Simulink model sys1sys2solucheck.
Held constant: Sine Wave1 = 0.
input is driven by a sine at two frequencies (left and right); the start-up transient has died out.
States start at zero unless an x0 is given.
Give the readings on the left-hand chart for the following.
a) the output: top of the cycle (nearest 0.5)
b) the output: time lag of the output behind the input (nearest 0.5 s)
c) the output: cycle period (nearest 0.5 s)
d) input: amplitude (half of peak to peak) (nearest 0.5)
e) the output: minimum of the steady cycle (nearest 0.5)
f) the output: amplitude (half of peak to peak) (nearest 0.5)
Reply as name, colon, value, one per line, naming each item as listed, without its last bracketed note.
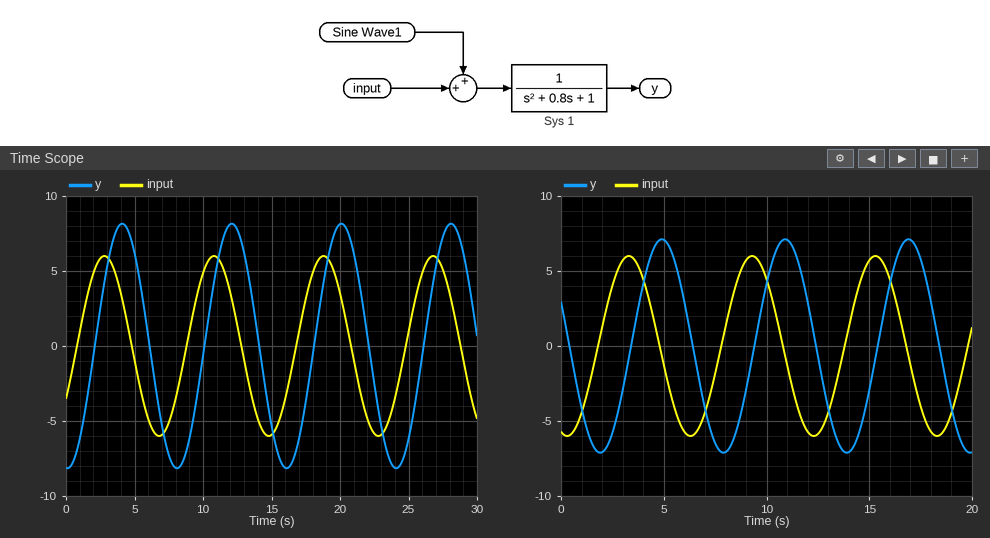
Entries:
the output: top of the cycle: 8.0
the output: time lag of the output behind the input: 1.5 s
the output: cycle period: 8.0 s
input: amplitude (half of peak to peak): 6.0
the output: minimum of the steady cycle: -8.0
the output: amplitude (half of peak to peak): 8.0
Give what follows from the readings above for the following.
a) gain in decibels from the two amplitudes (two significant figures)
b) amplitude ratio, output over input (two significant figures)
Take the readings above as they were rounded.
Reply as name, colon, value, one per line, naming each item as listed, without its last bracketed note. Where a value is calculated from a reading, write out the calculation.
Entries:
gain in decibels from the two amplitudes: 20 log10(8 / 6) = 2.5 dB
amplitude ratio, output over input: 8 / 6 = 1.3
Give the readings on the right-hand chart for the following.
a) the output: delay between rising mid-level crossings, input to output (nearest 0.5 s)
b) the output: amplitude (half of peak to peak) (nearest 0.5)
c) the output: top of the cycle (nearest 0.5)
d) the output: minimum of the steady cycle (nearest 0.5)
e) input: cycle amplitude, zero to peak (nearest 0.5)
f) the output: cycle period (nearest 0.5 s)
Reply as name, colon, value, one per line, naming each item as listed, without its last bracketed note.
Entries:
the output: delay between rising mid-level crossings, input to output: 1.5 s
the output: amplitude (half of peak to peak): 7.0
the output: top of the cycle: 7.0
the output: minimum of the steady cycle: -7.0
input: cycle amplitude, zero to peak: 6.0
the output: cycle period: 6.0 s
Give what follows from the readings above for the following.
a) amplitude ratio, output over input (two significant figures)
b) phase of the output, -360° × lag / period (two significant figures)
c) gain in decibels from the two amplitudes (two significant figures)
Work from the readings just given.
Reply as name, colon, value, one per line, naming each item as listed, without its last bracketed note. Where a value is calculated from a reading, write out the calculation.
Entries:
amplitude ratio, output over input: 7 / 6 = 1.2
phase of the output, -360° × lag / period: -360 × 1.5 / 6 = -90°
gain in decibels from the two amplitudes: 20 log10(7 / 6) = 1.3 dB
